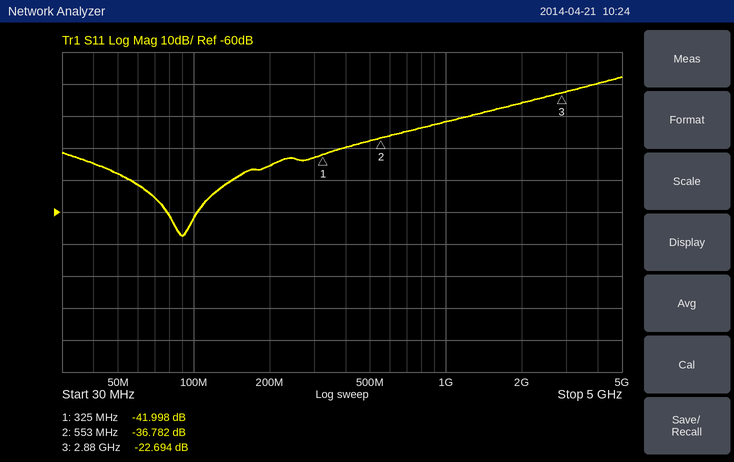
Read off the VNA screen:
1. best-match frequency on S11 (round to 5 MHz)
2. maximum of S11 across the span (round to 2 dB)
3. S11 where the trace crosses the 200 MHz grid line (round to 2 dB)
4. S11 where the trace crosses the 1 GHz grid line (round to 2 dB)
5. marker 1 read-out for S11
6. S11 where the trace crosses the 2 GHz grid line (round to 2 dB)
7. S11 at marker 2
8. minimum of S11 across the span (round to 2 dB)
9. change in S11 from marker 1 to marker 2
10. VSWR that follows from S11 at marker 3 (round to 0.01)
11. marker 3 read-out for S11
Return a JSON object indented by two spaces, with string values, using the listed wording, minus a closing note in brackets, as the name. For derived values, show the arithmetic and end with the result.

{
  "best-match frequency on S11": "90 MHz",
  "maximum of S11 across the span": "-18 dB",
  "S11 where the trace crosses the 200 MHz grid line": "-46 dB",
  "S11 where the trace crosses the 1 GHz grid line": "-32 dB",
  "marker 1 read-out for S11": "-41.998 dB",
  "S11 where the trace crosses the 2 GHz grid line": "-26 dB",
  "S11 at marker 2": "-36.782 dB",
  "minimum of S11 across the span": "-68 dB",
  "change in S11 from marker 1 to marker 2": "-36.782 − (-41.998) = 5.216 dB",
  "VSWR that follows from S11 at marker 3": "(1 + 0.0733)/(1 − 0.0733) ≈ 1.16",
  "marker 3 read-out for S11": "-22.694 dB"
}
